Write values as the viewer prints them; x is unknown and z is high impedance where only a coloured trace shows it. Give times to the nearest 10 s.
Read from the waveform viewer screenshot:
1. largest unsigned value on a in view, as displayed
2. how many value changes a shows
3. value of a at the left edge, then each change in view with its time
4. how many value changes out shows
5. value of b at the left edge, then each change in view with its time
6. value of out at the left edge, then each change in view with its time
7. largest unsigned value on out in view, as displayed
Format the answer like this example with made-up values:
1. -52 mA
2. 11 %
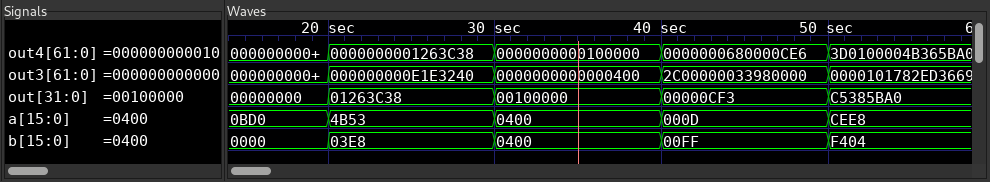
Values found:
1. CEE8
2. 4
3. 0BD0, 4B53 at 20 s, 0400 at 30 s, 000D at 40 s, CEE8 at 50 s
4. 4
5. 0000, 03E8 at 20 s, 0400 at 30 s, 00FF at 40 s, F404 at 50 s
6. 00000000, 01263C38 at 20 s, 00100000 at 30 s, 00000CF3 at 40 s, C5385BA0 at 50 s
7. C5385BA0
